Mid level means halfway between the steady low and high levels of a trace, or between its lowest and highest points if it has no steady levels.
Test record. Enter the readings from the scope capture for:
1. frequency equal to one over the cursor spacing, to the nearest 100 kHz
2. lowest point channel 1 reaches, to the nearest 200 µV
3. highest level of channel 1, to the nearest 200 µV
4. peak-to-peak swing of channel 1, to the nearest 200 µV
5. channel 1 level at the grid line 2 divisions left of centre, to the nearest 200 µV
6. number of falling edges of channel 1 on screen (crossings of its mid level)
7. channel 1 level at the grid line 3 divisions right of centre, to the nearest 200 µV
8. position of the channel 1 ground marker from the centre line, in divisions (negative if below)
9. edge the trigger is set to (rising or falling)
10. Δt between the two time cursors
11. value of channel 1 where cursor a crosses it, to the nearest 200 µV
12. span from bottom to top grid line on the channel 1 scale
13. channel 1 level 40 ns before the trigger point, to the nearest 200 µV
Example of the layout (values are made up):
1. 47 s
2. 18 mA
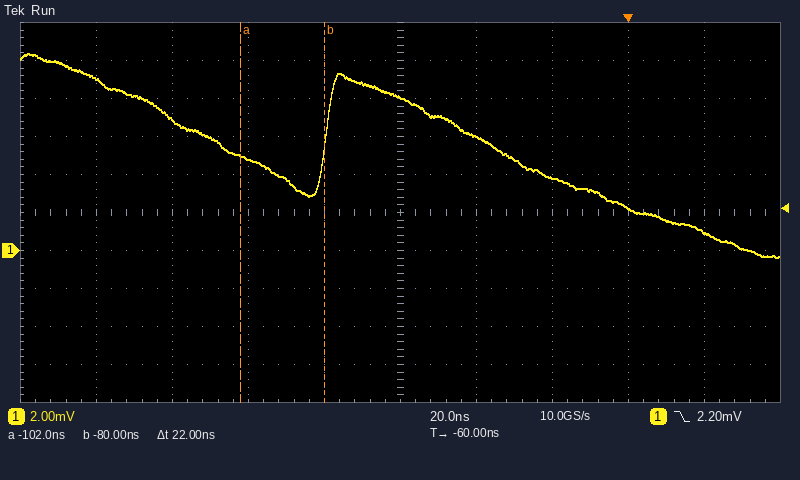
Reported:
1. 45.5 MHz
2. -400 µV
3. 10.4 mV
4. 10.8 mV
5. 4.8 mV
6. 2
7. 2.2 mV
8. -1.0 div
9. falling
10. 22 ns
11. 5.0 mV
12. 20 mV
13. 6.0 mV
